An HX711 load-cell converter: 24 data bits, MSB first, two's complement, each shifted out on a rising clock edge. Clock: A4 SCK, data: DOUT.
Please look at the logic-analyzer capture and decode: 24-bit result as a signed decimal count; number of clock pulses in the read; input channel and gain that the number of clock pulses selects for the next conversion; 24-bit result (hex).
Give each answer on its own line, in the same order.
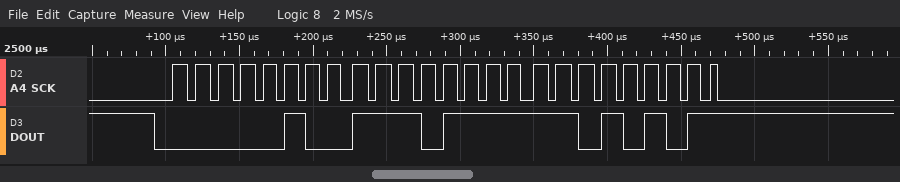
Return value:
323541
25
channel A, gain 128
0x04EFD5
